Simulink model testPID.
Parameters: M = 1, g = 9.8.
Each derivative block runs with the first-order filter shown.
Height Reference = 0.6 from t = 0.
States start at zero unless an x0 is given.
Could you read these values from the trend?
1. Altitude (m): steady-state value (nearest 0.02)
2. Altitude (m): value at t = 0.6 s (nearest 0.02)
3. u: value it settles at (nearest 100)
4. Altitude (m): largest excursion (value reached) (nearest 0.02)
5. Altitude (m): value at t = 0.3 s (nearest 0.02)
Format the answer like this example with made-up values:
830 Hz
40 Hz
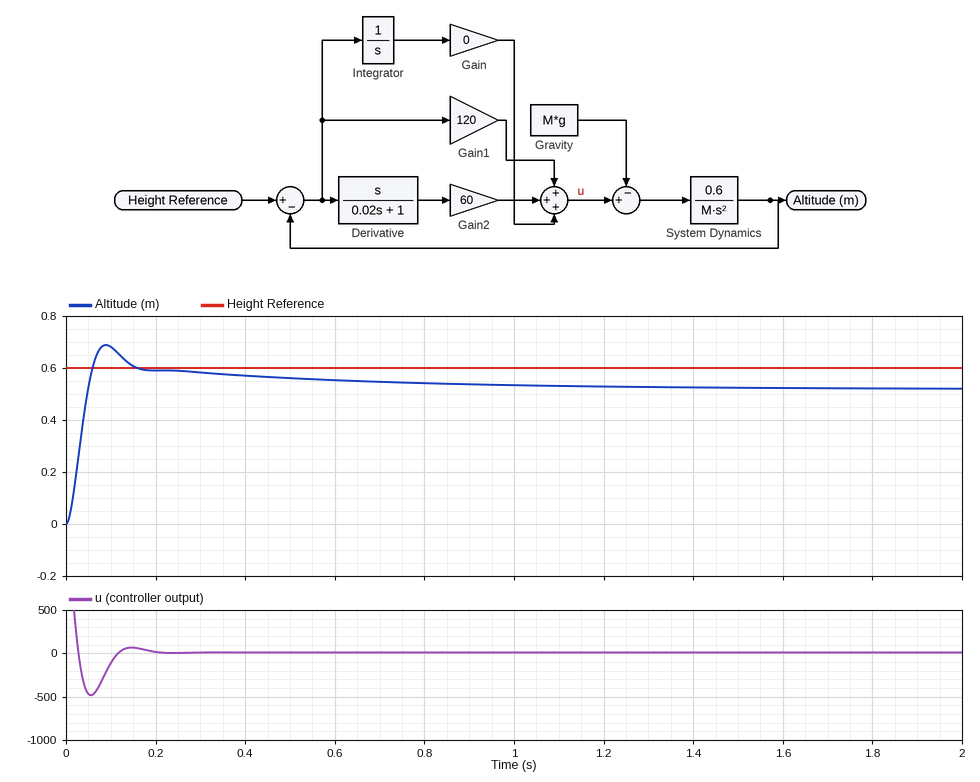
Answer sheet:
0.52
0.56
0
0.68
0.58
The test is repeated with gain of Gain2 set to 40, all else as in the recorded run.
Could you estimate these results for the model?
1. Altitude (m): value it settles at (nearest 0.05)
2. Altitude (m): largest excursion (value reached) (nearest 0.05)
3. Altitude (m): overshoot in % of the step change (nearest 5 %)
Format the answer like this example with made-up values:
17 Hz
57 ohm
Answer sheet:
0.50
0.65
30 %
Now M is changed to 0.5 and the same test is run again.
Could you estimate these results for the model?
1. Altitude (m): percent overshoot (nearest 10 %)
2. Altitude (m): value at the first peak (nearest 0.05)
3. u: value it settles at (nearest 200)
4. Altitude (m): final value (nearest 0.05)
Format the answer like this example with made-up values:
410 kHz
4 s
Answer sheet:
40 %
0.75
0
0.55
